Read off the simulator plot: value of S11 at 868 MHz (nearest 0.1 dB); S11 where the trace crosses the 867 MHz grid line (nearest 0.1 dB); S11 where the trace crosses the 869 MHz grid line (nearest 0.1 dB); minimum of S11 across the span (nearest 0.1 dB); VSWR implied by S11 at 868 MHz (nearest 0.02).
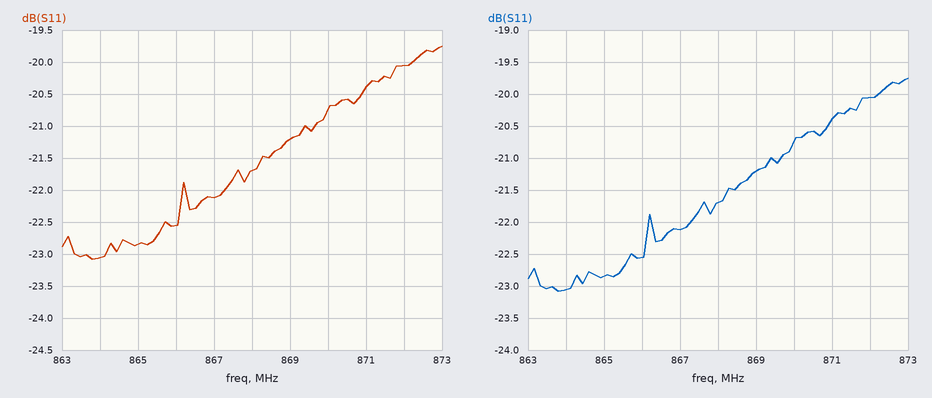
-21.7 dB
-22.1 dB
-21.2 dB
-23.1 dB
1.18
